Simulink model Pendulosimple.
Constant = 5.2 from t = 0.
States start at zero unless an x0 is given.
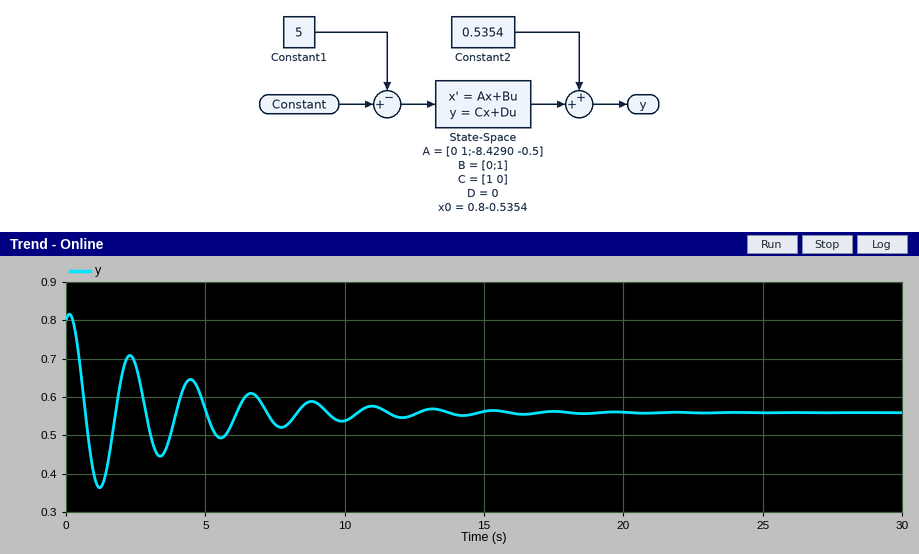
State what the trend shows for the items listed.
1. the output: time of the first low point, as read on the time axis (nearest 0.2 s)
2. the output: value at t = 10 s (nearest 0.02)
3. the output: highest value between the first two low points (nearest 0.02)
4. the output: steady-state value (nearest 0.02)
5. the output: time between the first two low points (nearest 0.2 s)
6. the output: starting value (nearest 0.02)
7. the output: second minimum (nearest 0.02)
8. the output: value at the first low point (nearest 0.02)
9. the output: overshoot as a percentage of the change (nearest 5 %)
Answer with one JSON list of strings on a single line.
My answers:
["1.2 s", "0.54", "0.70", "0.56", "2.2 s", "0.80", "0.44", "0.36", "80 %"]
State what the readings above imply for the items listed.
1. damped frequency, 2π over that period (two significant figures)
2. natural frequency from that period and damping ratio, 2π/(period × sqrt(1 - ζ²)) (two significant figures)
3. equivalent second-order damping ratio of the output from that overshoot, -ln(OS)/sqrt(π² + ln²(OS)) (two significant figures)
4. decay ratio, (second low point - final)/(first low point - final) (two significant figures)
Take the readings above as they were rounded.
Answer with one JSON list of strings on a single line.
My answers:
["2.9 rad/s", "2.9 rad/s", "0.071", "0.60"]
